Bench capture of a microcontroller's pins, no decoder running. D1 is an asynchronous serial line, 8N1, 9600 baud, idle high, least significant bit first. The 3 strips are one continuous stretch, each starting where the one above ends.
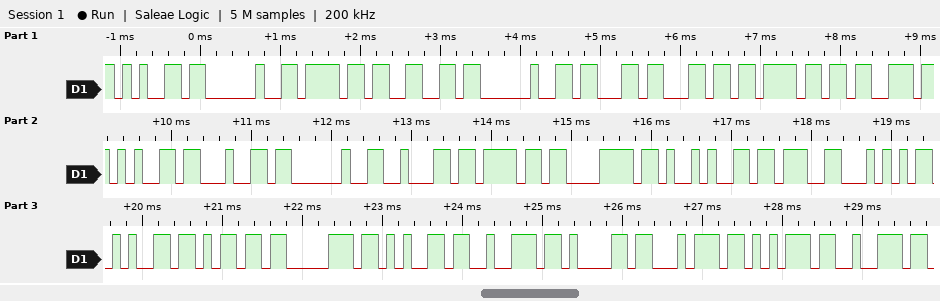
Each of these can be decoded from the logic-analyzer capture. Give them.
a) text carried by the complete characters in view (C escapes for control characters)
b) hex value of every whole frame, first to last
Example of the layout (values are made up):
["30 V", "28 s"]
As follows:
["\"e of closed box);Temperatur\"", "0x65 0x20 0x6F 0x66 0x20 0x63 0x6C 0x6F 0x73 0x65 0x64 0x20 0x62 0x6F 0x78 0x29 0x3B 0x54 0x65 0x6D 0x70 0x65 0x72 0x61 0x74 0x75 0x72"]
